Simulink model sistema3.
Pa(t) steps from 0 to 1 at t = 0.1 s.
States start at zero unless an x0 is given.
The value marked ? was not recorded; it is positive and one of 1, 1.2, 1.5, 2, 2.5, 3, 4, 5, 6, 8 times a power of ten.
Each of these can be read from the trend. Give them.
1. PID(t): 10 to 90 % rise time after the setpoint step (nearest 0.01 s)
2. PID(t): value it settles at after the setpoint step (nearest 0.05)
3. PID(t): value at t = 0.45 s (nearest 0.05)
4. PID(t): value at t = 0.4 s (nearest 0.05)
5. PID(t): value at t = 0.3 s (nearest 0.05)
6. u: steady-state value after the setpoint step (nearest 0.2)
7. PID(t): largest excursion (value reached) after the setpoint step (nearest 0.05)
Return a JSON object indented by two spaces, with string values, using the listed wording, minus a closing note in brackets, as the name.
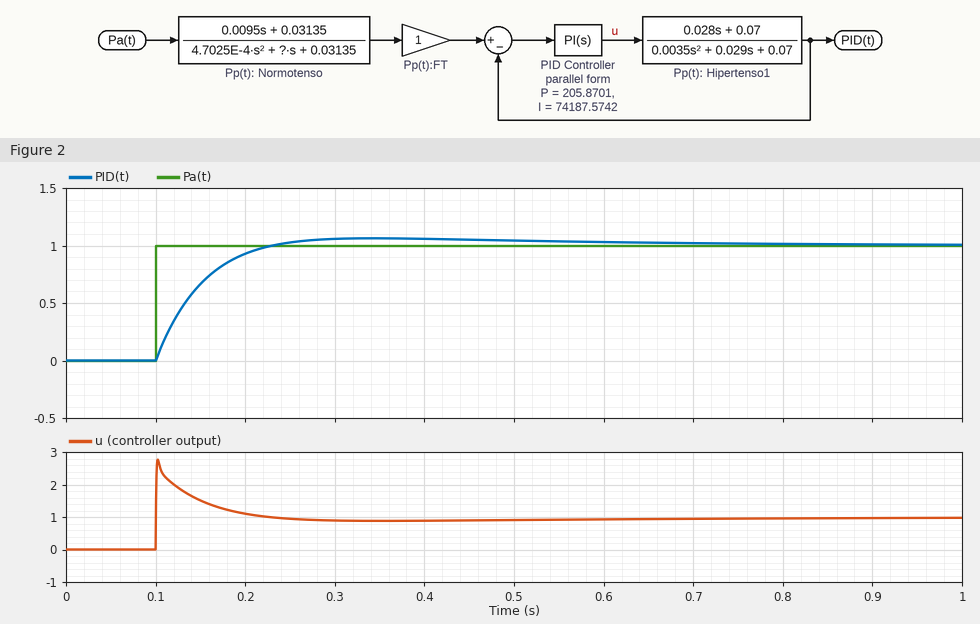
{
  "PID(t): 10 to 90 % rise time after the setpoint step": "0.09 s",
  "PID(t): value it settles at after the setpoint step": "1.00",
  "PID(t): value at t = 0.45 s": "1.05",
  "PID(t): value at t = 0.4 s": "1.05",
  "PID(t): value at t = 0.3 s": "1.05",
  "u: steady-state value after the setpoint step": "1.0",
  "PID(t): largest excursion (value reached) after the setpoint step": "1.05"
}
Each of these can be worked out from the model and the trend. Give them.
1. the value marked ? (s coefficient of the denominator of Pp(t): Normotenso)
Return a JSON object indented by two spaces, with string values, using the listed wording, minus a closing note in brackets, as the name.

{
  "the value marked ? (s coefficient of the denominator of Pp(t): Normotenso)": "0.01"
}
